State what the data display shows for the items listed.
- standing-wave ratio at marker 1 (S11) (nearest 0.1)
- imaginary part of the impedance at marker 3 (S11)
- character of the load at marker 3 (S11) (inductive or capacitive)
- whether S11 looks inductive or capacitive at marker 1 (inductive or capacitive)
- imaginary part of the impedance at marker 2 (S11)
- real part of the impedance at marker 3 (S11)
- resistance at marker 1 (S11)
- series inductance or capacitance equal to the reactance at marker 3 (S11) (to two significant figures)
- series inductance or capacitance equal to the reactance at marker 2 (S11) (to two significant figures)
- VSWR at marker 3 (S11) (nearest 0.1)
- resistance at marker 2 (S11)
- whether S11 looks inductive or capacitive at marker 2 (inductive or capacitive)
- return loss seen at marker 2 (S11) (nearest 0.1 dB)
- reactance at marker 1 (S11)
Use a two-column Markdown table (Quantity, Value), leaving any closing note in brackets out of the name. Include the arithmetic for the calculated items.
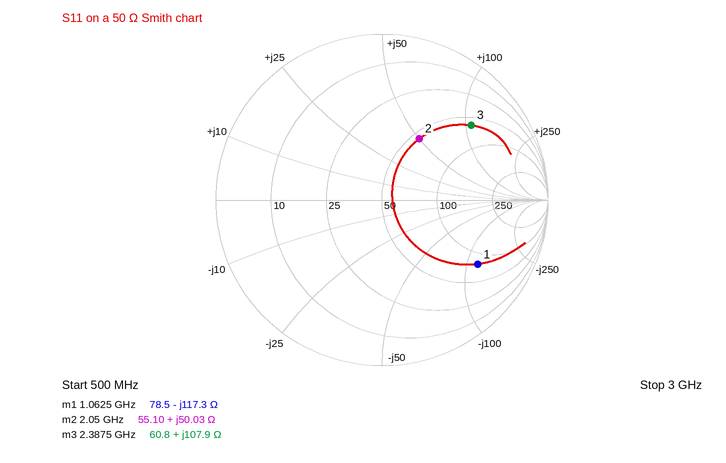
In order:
| Quantity | Value |
|---|---|
| standing-wave ratio at marker 1 (S11) | 5.5 |
| imaginary part of the impedance at marker 3 | +107.9 Ω |
| character of the load at marker 3 (S11) | inductive |
| whether S11 looks inductive or capacitive at marker 1 | capacitive |
| imaginary part of the impedance at marker 2 | +50.03 Ω |
| real part of the impedance at marker 3 | 60.8 Ω |
| resistance at marker 1 | 78.5 Ω |
| series inductance or capacitance equal to the reactance at marker 3 (S11) | L = 107.9 Ω/(2π × 2.3875 GHz) ≈ 7.2 nH |
| series inductance or capacitance equal to the reactance at marker 2 (S11) | L = 50.03 Ω/(2π × 2.05 GHz) ≈ 3.9 nH |
| VSWR at marker 3 (S11) | 5.7 |
| resistance at marker 2 | 55.10 Ω |
| whether S11 looks inductive or capacitive at marker 2 | inductive |
| return loss seen at marker 2 (S11) | 7.3 dB |
| reactance at marker 1 | -117.3 Ω |
